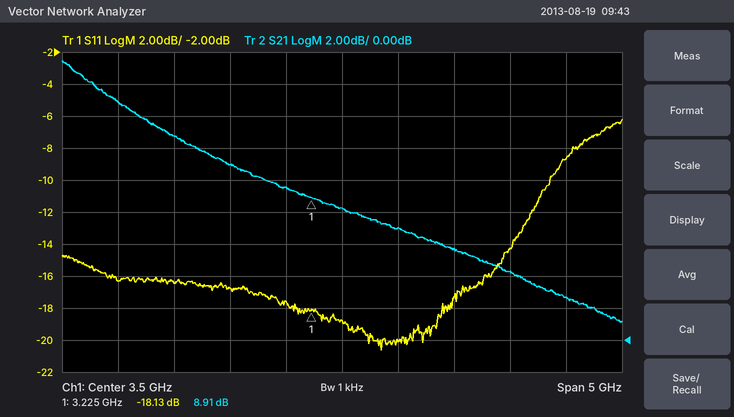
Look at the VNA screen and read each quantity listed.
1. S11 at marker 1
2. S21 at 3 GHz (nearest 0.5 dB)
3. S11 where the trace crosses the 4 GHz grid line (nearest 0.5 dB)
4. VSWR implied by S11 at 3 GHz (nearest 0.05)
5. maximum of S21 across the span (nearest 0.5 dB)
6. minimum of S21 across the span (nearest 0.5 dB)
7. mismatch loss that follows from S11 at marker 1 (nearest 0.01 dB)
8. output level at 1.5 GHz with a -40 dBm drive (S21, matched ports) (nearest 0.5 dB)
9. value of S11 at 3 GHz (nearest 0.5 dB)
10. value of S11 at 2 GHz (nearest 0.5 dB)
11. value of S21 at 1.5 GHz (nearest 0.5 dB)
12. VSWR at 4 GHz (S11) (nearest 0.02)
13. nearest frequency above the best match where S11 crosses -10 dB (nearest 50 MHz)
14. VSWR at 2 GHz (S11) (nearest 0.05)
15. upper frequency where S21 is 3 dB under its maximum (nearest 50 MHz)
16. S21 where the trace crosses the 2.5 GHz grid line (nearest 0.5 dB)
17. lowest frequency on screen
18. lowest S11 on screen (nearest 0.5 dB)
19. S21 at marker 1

-18.13 dB
9.5 dB
-20.0 dB
1.30
17.5 dB
1.0 dB
0.07 dB
-25.0 dBm
-17.5 dB
-16.5 dB
15.0 dB
1.22
5.35 GHz
1.35
1.60 GHz
11.0 dB
1 GHz
-20.5 dB
8.91 dB
